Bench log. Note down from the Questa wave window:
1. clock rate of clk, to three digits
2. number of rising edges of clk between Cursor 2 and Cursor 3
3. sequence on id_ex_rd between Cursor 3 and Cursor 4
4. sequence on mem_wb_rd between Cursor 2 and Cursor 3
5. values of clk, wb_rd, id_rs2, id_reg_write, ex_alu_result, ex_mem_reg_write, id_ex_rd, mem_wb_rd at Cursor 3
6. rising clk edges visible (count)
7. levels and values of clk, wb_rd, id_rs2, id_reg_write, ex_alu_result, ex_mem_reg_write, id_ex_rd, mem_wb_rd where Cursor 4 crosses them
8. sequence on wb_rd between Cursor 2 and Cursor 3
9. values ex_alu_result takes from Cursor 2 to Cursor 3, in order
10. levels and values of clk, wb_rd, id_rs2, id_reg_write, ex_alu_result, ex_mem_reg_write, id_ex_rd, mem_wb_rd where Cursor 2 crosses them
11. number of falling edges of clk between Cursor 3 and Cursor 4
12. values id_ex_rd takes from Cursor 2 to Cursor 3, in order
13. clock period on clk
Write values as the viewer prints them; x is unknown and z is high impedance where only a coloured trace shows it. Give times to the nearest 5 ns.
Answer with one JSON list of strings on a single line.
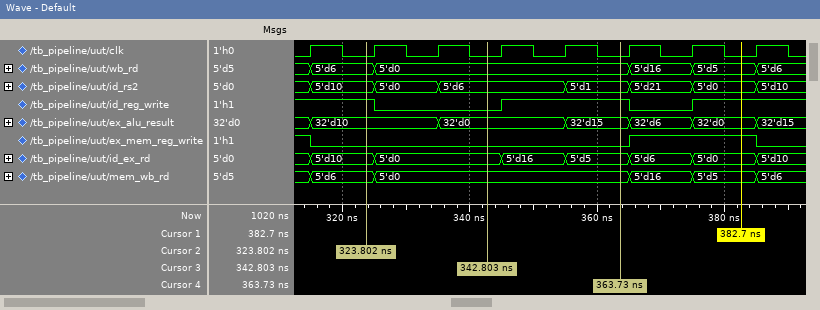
["100 MHz", "2", "5'd0, 5'd16, 5'd5", "5'd6, 5'd0", "clk=0, wb_rd=5'd0, id_rs2=5'd6, id_reg_write=0, ex_alu_result=32'd0, ex_mem_reg_write=0, id_ex_rd=5'd0, mem_wb_rd=5'd0", "8", "clk=0, wb_rd=5'd0, id_rs2=5'd1, id_reg_write=1, ex_alu_result=32'd15, ex_mem_reg_write=0, id_ex_rd=5'd5, mem_wb_rd=5'd0", "5'd6, 5'd0", "32'd10, 32'd0", "clk=0, wb_rd=5'd6, id_rs2=5'd10, id_reg_write=1, ex_alu_result=32'd10, ex_mem_reg_write=0, id_ex_rd=5'd10, mem_wb_rd=5'd6", "2", "5'd10, 5'd0", "10 ns"]
